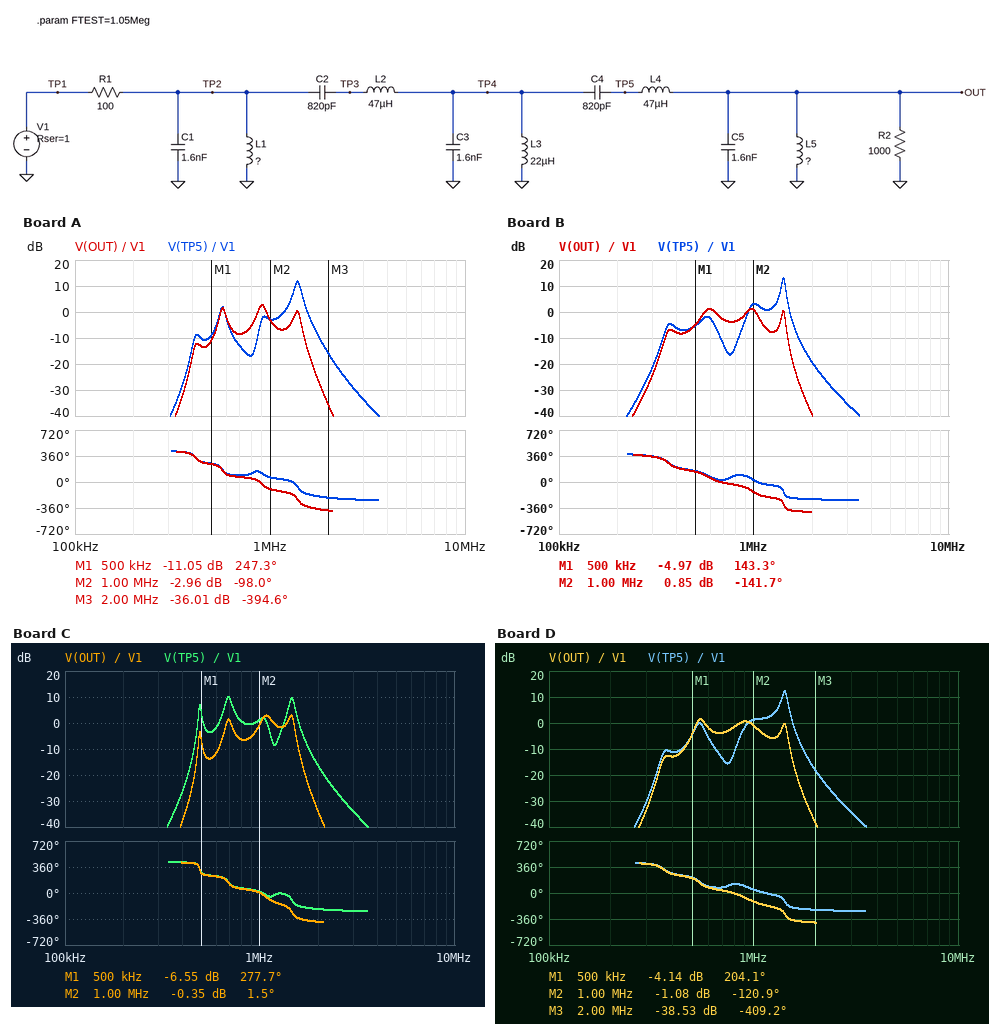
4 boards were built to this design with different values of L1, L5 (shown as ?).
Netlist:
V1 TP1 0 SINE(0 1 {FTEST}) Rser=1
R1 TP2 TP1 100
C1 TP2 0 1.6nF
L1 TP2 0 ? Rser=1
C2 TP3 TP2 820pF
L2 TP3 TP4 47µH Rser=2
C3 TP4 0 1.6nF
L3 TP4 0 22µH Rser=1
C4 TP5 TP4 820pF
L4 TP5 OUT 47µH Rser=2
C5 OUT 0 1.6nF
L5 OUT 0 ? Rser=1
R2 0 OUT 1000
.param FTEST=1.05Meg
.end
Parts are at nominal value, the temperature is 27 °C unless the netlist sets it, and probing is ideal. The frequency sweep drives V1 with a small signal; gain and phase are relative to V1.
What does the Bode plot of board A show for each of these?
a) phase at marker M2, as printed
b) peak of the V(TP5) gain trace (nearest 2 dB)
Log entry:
-98.0 deg
12 dB
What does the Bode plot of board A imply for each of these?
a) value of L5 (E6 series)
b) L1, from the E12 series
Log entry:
47 µH
8.2 µH
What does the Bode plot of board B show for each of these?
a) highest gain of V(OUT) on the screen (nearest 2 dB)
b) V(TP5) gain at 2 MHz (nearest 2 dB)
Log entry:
2 dB
-20 dB
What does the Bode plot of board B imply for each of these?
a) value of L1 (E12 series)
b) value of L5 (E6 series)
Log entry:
68 µH
68 µH
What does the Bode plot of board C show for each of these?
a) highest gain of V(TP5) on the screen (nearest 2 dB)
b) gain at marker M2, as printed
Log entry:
10 dB
-0.35 dB
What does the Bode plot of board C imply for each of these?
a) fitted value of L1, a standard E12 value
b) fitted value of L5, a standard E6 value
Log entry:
10 µH
15 µH
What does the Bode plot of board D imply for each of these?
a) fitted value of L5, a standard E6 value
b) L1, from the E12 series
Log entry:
68 µH
18 µH
